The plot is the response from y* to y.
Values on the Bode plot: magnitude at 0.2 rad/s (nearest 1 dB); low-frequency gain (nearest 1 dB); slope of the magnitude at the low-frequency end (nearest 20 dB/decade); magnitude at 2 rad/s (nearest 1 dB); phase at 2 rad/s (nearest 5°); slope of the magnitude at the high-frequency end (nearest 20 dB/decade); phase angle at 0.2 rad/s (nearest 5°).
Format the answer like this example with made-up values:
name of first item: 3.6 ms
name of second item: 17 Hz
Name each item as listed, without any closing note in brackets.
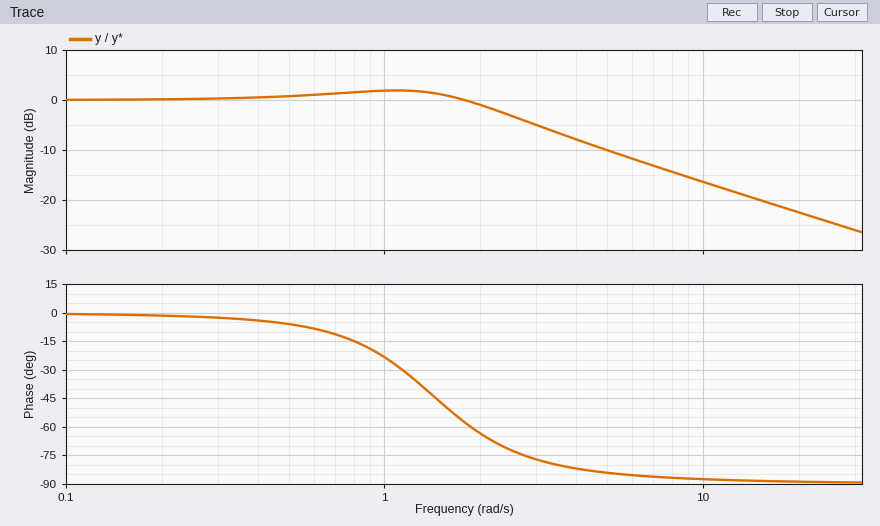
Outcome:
magnitude at 0.2 rad/s: 0 dB
low-frequency gain: 0 dB
slope of the magnitude at the low-frequency end: 0 dB/decade
magnitude at 2 rad/s: -1 dB
phase at 2 rad/s: -65°
slope of the magnitude at the high-frequency end: -20 dB/decade
phase angle at 0.2 rad/s: 0°
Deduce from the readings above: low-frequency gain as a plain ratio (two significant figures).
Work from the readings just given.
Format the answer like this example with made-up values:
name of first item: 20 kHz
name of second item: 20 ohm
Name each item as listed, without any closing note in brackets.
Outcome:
low-frequency gain as a plain ratio: 1.0
